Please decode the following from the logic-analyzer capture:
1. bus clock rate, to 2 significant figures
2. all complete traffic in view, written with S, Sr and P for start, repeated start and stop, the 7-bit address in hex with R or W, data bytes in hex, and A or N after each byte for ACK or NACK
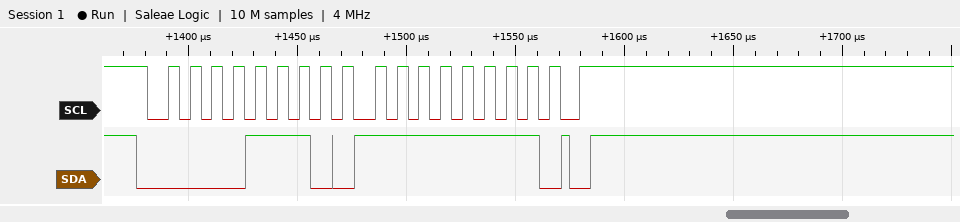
100 kHz
S 07W A FF A P
